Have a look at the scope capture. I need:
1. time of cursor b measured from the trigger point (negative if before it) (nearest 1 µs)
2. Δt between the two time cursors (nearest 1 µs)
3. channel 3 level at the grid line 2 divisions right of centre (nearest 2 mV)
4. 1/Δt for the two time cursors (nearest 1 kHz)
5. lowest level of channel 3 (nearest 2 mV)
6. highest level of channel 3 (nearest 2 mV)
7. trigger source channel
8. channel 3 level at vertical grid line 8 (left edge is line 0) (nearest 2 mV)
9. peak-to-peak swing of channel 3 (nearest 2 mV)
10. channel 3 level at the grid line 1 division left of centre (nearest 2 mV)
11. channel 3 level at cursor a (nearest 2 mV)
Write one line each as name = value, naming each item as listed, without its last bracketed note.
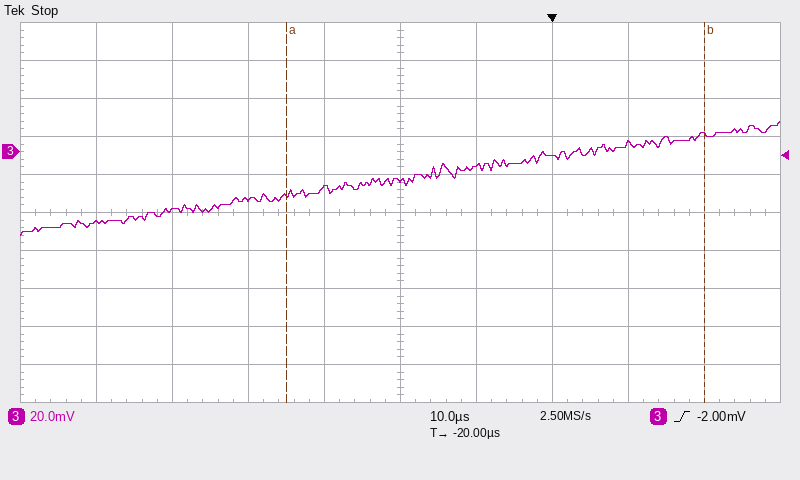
time of cursor b measured from the trigger point (negative if before it) = +20 µs
Δt between the two time cursors = 55 µs
channel 3 level at the grid line 2 divisions right of centre = -2 mV
1/Δt for the two time cursors = 18 kHz
lowest level of channel 3 = -44 mV
highest level of channel 3 = 16 mV
trigger source channel = channel 3
channel 3 level at vertical grid line 8 (left edge is line 0) = 4 mV
peak-to-peak swing of channel 3 = 60 mV
channel 3 level at the grid line 1 division left of centre = -20 mV
channel 3 level at cursor a = -22 mV
